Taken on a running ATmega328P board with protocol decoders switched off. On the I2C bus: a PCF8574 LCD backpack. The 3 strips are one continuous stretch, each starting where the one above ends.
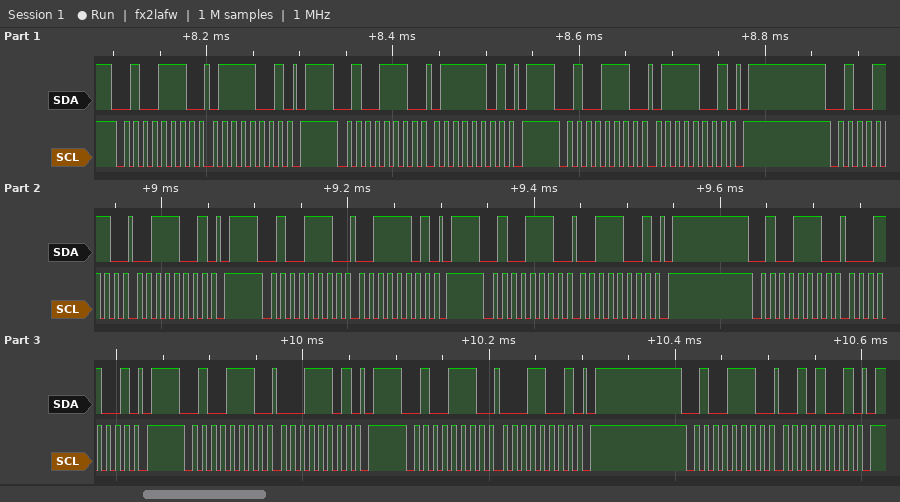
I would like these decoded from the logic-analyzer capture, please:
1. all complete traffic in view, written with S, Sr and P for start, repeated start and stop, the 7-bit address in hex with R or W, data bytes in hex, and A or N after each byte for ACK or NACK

S 27W A 79 A P S 27W A 7D A P S 27W A 79 A P S 27W A 39 A P S 27W A 3D A P S 27W A 39 A P S 27W A 19 A P S 27W A 1D A P S 27W A 19 A P S 27W A 29 A P
